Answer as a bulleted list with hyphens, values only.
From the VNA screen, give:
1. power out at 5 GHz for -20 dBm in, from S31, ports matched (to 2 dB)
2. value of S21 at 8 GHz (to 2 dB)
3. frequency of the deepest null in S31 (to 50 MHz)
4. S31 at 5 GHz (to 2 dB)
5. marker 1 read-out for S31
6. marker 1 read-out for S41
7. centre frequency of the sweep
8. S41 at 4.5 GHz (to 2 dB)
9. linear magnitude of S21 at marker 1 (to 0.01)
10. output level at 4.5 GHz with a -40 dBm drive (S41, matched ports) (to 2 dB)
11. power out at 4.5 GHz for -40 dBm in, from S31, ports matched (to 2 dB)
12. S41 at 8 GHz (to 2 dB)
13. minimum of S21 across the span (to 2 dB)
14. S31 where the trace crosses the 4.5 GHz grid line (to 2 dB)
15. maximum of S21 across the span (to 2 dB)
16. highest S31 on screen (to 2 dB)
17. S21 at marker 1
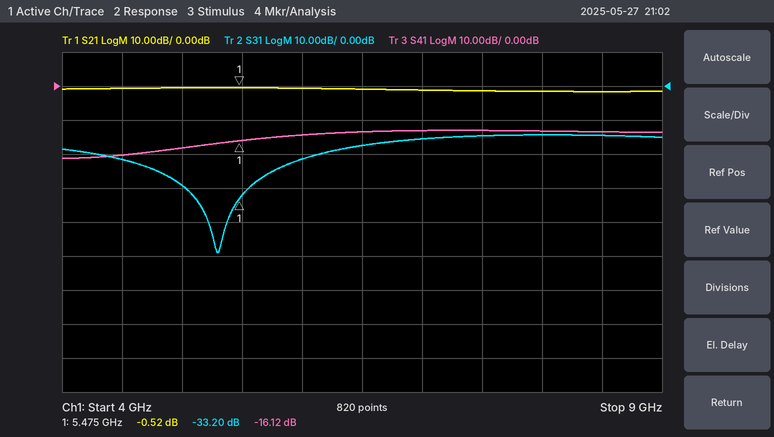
- -50 dBm
- -2 dB
- 5.30 GHz
- -30 dB
- -33.20 dB
- -16.12 dB
- 6.5 GHz
- -20 dB
- 0.94
- -60 dBm
- -62 dBm
- -14 dB
- -2 dB
- -22 dB
- 0 dB
- -14 dB
- -0.52 dB
